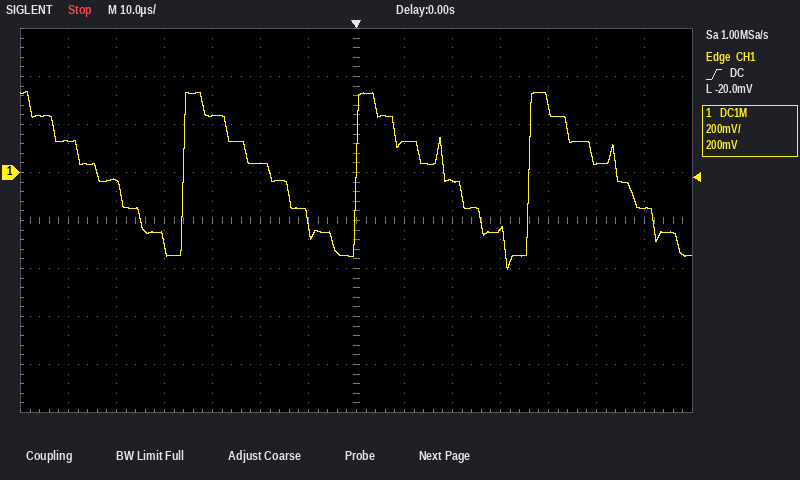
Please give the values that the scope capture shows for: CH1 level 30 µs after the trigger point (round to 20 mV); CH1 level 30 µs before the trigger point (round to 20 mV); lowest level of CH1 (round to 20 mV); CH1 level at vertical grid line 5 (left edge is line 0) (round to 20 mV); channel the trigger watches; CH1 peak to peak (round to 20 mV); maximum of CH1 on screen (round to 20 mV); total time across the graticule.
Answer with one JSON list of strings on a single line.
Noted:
["-240 mV", "240 mV", "-400 mV", "40 mV", "CH1", "740 mV", "340 mV", "140 µs"]
